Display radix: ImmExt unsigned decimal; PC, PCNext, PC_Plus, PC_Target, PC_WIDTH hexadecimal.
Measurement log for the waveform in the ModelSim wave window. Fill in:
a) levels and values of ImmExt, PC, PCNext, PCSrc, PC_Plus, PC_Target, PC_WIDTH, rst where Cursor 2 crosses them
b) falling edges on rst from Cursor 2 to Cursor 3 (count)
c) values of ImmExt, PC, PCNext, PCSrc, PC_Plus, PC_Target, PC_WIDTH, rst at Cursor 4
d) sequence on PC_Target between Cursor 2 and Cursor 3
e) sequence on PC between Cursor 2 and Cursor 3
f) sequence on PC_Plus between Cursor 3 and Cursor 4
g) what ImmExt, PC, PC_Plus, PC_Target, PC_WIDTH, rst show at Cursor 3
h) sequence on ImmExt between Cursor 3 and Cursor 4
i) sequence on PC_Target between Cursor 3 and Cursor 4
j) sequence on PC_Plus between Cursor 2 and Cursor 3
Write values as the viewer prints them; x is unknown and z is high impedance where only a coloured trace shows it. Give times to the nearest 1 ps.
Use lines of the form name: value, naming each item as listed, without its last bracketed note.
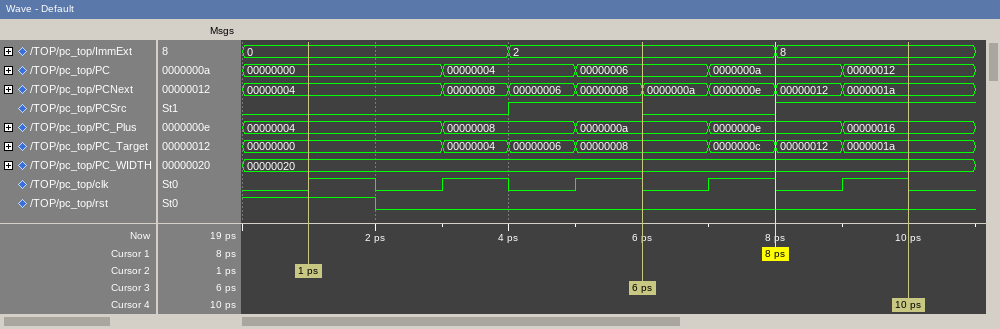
levels and values of ImmExt, PC, PCNext, PCSrc, PC_Plus, PC_Target, PC_WIDTH, rst where Cursor 2 crosses them: ImmExt=0, PC=00000000, PCNext=00000004, PCSrc=0, PC_Plus=00000004, PC_Target=00000000, PC_WIDTH=00000020, rst=1
falling edges on rst from Cursor 2 to Cursor 3: 1
values of ImmExt, PC, PCNext, PCSrc, PC_Plus, PC_Target, PC_WIDTH, rst at Cursor 4: ImmExt=8, PC=00000012, PCNext=0000001a, PCSrc=1, PC_Plus=00000016, PC_Target=0000001a, PC_WIDTH=00000020, rst=0
sequence on PC_Target between Cursor 2 and Cursor 3: 00000000, 00000004, 00000006, 00000008
sequence on PC between Cursor 2 and Cursor 3: 00000000, 00000004, 00000006
sequence on PC_Plus between Cursor 3 and Cursor 4: 0000000a, 0000000e, 00000016
what ImmExt, PC, PC_Plus, PC_Target, PC_WIDTH, rst show at Cursor 3: ImmExt=2, PC=00000006, PC_Plus=0000000a, PC_Target=00000008, PC_WIDTH=00000020, rst=0
sequence on ImmExt between Cursor 3 and Cursor 4: 2, 8
sequence on PC_Target between Cursor 3 and Cursor 4: 00000008, 0000000c, 00000012, 0000001a
sequence on PC_Plus between Cursor 2 and Cursor 3: 00000004, 00000008, 0000000a
